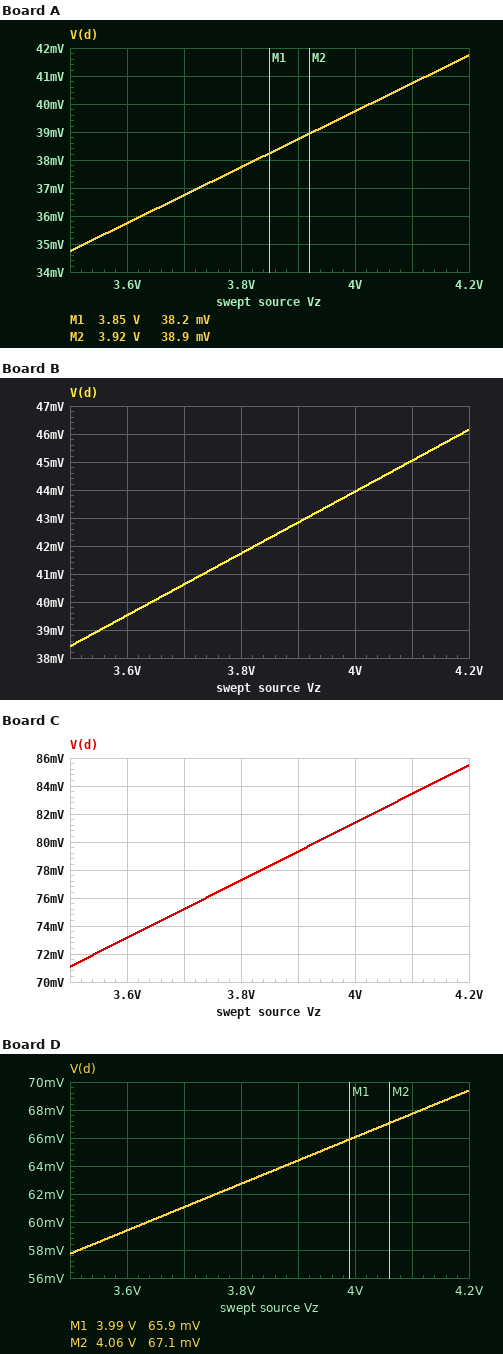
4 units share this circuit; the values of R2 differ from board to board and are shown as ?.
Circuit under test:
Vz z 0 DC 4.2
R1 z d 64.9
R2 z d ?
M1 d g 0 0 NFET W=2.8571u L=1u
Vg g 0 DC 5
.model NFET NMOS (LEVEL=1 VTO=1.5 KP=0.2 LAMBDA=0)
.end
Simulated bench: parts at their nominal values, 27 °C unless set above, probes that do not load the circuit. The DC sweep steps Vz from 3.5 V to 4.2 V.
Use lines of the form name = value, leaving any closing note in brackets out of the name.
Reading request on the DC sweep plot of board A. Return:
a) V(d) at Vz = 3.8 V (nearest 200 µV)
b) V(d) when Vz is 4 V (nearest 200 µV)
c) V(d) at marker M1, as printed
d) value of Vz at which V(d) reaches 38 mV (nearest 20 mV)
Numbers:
V(d) at Vz = 3.8 V = 37.8 mV
V(d) when Vz is 4 V = 39.8 mV
V(d) at marker M1, as printed = 38.2 mV
value of Vz at which V(d) reaches 38 mV = 3.82 V
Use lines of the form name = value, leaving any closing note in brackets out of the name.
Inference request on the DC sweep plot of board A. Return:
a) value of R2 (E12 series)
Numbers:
value of R2 = 220 Ω
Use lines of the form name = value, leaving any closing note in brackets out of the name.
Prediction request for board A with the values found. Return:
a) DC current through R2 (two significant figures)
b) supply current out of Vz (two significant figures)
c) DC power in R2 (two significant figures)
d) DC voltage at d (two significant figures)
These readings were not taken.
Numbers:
DC current through R2 = 19 mA
supply current out of Vz = 83 mA
DC power in R2 = 79 mW
DC voltage at d = 42 mV
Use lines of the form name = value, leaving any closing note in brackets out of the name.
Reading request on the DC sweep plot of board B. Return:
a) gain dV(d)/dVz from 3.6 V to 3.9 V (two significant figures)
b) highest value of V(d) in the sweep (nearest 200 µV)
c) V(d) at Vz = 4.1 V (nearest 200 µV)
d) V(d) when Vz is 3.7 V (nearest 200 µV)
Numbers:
gain dV(d)/dVz from 3.6 V to 3.9 V = 0.011 V/V
highest value of V(d) in the sweep = 46.2 mV
V(d) at Vz = 4.1 V = 45.0 mV
V(d) when Vz is 3.7 V = 40.6 mV
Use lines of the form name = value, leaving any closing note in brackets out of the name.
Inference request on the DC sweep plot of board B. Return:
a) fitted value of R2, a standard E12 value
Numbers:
fitted value of R2, a standard E12 value = 150 Ω
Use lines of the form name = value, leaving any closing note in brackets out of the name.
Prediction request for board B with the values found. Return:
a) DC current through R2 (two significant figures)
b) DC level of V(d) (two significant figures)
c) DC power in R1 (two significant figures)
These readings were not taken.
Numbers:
DC current through R2 = 28 mA
DC level of V(d) = 46 mV
DC power in R1 = 270 mW
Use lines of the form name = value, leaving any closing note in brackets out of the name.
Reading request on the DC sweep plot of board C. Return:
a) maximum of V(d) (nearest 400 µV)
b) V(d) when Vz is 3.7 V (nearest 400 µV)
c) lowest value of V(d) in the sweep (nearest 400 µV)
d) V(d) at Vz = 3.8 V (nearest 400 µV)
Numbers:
maximum of V(d) = 85.6 mV
V(d) when Vz is 3.7 V = 75.2 mV
lowest value of V(d) in the sweep = 71.2 mV
V(d) at Vz = 3.8 V = 77.2 mV
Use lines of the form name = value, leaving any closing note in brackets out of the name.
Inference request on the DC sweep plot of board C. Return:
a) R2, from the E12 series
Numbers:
R2, from the E12 series = 39 Ω
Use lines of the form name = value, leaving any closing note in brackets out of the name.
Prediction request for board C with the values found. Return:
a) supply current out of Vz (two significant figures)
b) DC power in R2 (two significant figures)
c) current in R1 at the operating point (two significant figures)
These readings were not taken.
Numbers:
supply current out of Vz = 170 mA
DC power in R2 = 430 mW
current in R1 at the operating point = 63 mA
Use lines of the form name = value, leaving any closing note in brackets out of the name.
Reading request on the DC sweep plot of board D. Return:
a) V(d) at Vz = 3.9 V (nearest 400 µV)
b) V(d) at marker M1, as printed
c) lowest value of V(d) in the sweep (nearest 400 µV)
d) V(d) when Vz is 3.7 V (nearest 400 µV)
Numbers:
V(d) at Vz = 3.9 V = 64.4 mV
V(d) at marker M1, as printed = 65.9 mV
lowest value of V(d) in the sweep = 57.6 mV
V(d) when Vz is 3.7 V = 61.2 mV
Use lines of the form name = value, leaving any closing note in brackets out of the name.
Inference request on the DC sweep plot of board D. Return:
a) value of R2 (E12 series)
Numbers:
value of R2 = 56 Ω
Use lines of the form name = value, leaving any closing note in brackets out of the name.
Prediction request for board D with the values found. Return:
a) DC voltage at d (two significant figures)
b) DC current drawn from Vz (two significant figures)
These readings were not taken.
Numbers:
DC voltage at d = 69 mV
DC current drawn from Vz = 140 mA
